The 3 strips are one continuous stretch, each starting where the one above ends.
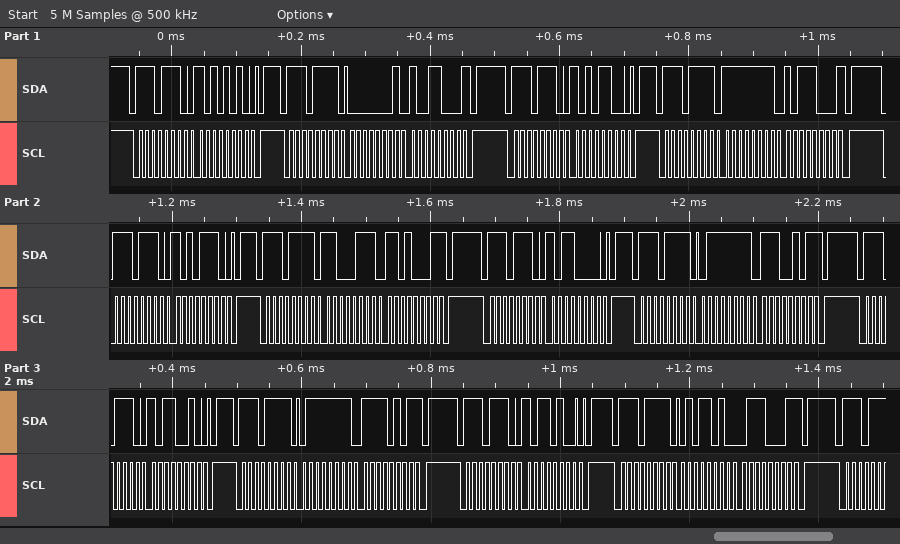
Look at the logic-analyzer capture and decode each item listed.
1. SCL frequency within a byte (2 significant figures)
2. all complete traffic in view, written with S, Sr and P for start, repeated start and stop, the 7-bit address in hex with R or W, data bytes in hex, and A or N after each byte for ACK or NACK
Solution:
100 kHz
S 77W A AA A P S 77R A 01 A 98 N P S 77W A AC A P S 77R A FF A B8 N P S 77W A AE A P S 77R A C7 A D1 N P S 77W A B0 A P S 77R A 7F A E5 N P S 77W A B2 A P S 77R A 7F A F5 N P S 77W A B4 A P S 77R A 5A A 71 N P
